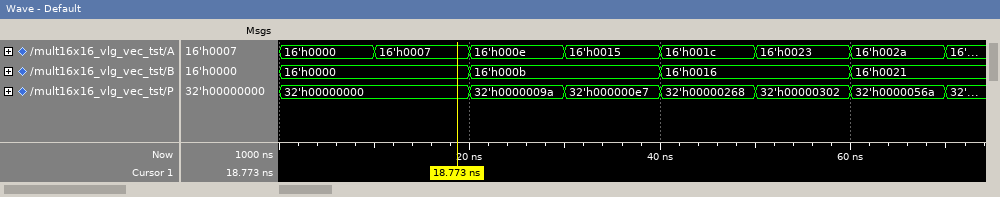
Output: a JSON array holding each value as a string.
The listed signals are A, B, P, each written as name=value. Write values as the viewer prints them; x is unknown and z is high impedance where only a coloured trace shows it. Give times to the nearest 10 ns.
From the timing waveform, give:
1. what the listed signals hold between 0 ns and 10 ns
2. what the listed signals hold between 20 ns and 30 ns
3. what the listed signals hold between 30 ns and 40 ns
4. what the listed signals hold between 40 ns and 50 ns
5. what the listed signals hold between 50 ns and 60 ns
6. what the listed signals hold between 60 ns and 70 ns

["A=16'h0000, B=16'h0000, P=32'h00000000", "A=16'h000e, B=16'h000b, P=32'h0000009a", "A=16'h0015, B=16'h000b, P=32'h000000e7", "A=16'h001c, B=16'h0016, P=32'h00000268", "A=16'h0023, B=16'h0016, P=32'h00000302", "A=16'h002a, B=16'h0021, P=32'h0000056a"]
